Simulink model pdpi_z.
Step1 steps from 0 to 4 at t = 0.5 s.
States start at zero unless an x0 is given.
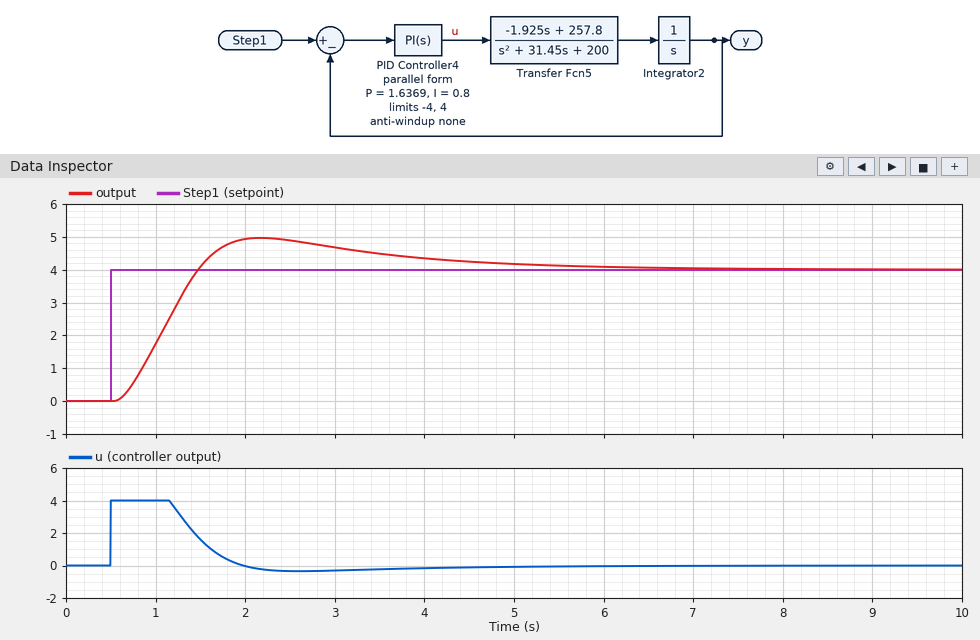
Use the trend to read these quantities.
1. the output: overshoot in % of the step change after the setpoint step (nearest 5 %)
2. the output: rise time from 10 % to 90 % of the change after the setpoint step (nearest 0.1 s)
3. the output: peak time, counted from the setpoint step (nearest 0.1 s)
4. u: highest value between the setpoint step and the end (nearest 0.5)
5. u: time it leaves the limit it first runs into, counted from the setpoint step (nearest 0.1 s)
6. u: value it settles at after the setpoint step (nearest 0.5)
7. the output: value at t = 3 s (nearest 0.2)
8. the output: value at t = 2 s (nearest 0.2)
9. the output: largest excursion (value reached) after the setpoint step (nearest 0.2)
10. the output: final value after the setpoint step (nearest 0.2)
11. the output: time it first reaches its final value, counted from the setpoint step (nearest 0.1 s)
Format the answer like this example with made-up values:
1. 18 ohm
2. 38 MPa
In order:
1. 25 %
2. 0.7 s
3. 1.7 s
4. 4.0
5. 0.7 s
6. 0.0
7. 4.6
8. 5.0
9. 5.0
10. 4.0
11. 1.0 s
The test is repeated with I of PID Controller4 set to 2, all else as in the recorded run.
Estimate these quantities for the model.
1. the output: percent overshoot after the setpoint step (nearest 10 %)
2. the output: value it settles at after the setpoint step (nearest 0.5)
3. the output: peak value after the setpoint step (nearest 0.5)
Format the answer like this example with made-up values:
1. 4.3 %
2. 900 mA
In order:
1. 50 %
2. 4.0
3. 6.0
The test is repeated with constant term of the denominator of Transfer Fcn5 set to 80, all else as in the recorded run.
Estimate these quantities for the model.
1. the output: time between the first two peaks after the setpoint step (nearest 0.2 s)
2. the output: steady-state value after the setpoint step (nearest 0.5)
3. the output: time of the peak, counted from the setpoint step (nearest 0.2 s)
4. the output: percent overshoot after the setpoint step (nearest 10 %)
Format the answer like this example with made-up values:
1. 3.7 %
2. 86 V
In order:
1. 1.8 s
2. 4.0
3. 1.0 s
4. 60 %
